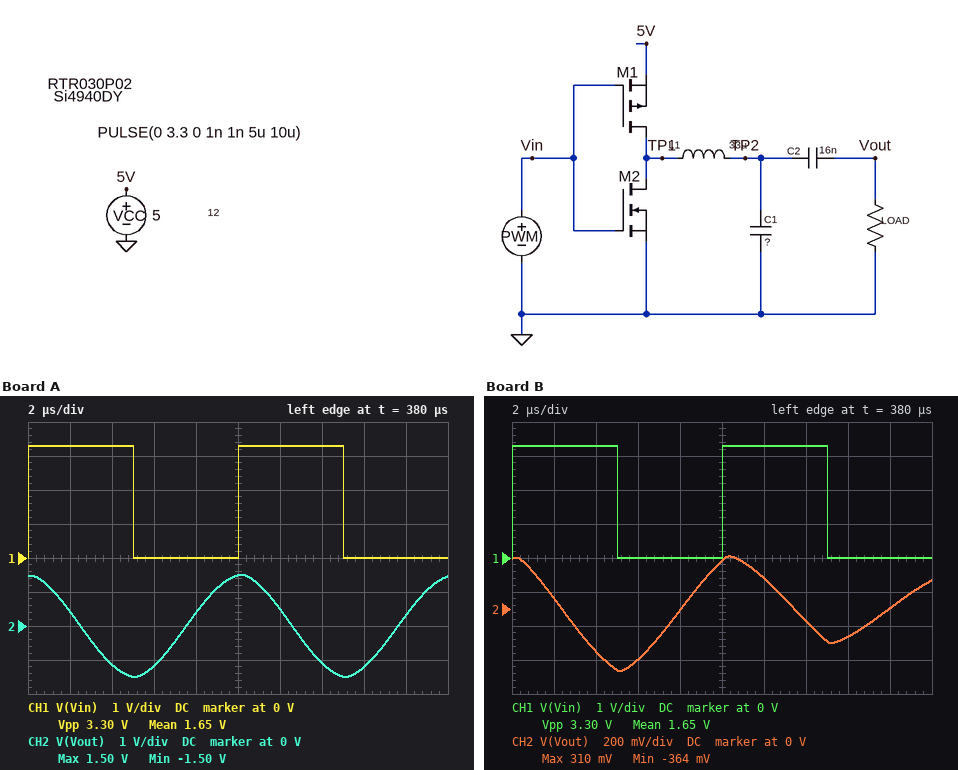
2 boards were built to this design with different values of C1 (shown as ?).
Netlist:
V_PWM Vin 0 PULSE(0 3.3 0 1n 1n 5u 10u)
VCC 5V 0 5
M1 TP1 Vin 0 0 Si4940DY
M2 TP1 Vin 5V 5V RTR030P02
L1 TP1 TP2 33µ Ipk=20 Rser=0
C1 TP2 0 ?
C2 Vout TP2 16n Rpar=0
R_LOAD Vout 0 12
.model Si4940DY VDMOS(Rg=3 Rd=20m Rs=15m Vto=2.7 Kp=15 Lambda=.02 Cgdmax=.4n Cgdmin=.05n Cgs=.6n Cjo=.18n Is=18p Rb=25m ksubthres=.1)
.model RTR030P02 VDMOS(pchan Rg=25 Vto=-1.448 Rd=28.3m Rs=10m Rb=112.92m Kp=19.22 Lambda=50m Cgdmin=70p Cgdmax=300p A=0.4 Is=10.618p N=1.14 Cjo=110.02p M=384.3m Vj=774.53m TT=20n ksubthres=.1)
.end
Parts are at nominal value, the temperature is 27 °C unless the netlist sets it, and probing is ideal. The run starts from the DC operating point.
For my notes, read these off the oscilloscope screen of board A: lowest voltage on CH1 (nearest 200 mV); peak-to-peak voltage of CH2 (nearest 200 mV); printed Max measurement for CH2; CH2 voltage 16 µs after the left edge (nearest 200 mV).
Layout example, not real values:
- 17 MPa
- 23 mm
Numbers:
- 0 V
- 3.0 V
- 1.50 V
- -1.2 V
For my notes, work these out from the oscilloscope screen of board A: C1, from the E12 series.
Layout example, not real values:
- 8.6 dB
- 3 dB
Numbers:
- 82 nF
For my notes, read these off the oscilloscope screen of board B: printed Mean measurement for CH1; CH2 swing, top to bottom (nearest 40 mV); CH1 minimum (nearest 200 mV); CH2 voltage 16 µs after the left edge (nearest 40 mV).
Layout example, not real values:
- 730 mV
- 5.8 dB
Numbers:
- 1.65 V
- 680 mV
- 0 V
- -160 mV
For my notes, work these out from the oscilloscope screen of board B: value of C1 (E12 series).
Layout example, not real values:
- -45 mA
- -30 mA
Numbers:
- 180 nF
